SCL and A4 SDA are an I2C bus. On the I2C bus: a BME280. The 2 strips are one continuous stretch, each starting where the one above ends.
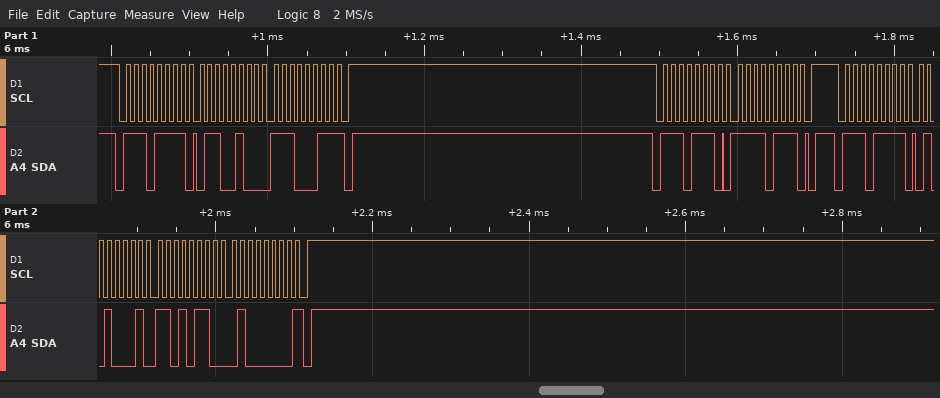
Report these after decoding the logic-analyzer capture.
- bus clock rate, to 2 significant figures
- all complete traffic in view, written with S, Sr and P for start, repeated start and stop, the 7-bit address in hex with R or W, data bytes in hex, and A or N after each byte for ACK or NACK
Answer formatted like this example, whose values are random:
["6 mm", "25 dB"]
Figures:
["100 kHz", "S 77R A 64 A E3 N P S 77W A F7 A P S 77R A 51 A D6 A 40 N P"]
